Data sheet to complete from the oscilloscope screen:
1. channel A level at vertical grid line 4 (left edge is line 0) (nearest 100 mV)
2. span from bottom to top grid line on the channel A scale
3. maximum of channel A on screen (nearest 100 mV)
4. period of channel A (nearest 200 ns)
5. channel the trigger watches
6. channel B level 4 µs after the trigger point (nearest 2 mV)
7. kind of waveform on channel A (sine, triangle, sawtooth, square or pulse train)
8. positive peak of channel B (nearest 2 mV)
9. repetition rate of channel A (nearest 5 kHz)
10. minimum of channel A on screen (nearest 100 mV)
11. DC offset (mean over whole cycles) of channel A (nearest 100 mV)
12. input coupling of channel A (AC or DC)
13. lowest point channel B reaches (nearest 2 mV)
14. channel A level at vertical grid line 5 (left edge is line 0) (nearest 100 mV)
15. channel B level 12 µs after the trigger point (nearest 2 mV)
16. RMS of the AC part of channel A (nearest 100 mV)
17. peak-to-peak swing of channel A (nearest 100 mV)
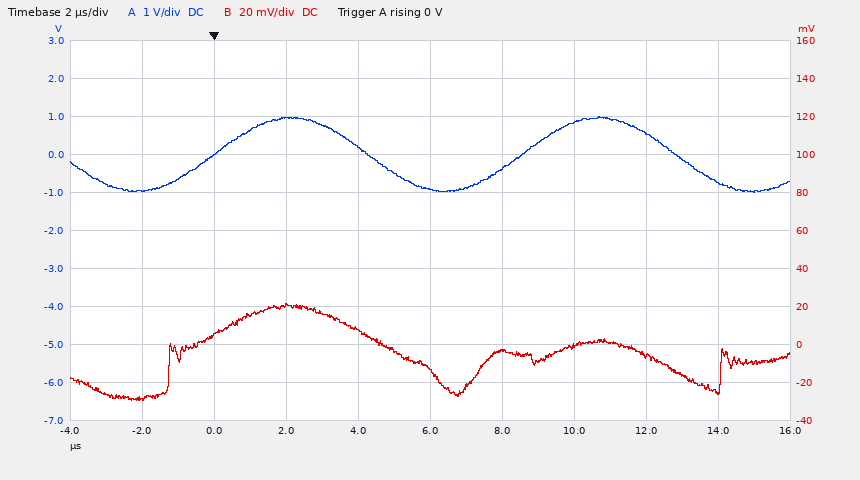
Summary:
200 mV
10 V
1.0 V
8.6 µs
channel A
8 mV
sine
22 mV
115 kHz
-1.0 V
0.0 V
DC
-30 mV
-900 mV
-6 mV
700 mV
2.0 V
